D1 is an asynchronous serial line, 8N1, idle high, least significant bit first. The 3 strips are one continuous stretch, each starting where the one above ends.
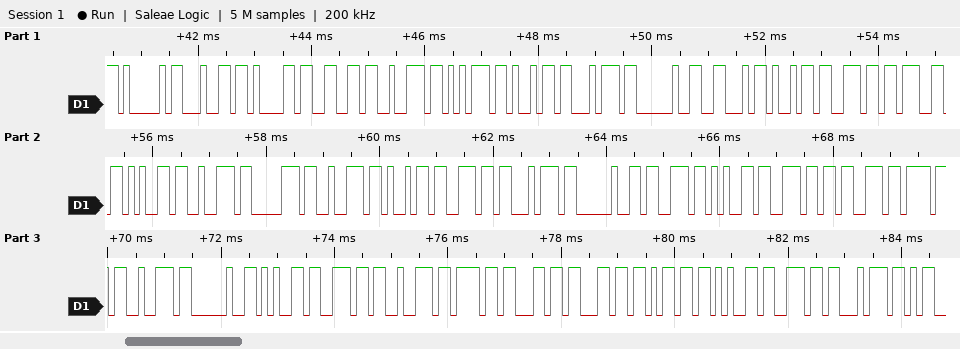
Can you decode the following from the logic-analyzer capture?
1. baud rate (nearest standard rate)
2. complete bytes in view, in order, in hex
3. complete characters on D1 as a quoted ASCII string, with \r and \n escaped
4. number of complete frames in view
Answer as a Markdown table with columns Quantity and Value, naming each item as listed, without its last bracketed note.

| Quantity | Value |
|---|---|
| baud rate | 9600 baud |
| complete bytes in view, in order, in hex | 41 64 61 66 72 75 69 74 20 46 69 6E 67 65 72 70 72 69 6E 74 20 73 65 6E 73 6F 72 20 65 6E 72 6F 6C 6C 6D 65 6E 74 |
| complete characters on D1 as a quoted ASCII string, with \r and \n escaped | "Adafruit Fingerprint sensor enrollment" |
| number of complete frames in view | 38 |
